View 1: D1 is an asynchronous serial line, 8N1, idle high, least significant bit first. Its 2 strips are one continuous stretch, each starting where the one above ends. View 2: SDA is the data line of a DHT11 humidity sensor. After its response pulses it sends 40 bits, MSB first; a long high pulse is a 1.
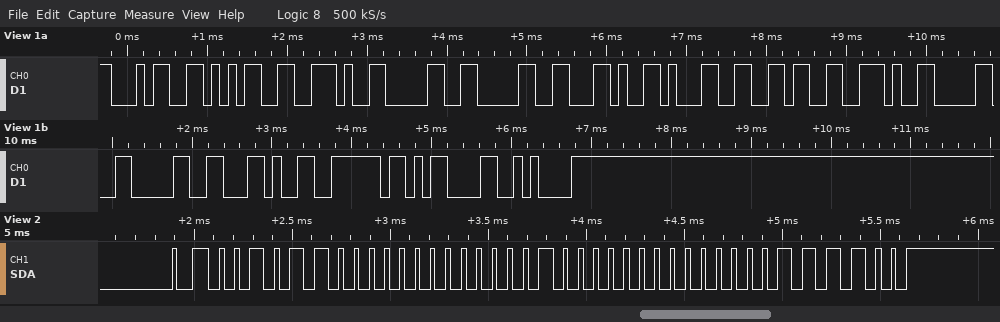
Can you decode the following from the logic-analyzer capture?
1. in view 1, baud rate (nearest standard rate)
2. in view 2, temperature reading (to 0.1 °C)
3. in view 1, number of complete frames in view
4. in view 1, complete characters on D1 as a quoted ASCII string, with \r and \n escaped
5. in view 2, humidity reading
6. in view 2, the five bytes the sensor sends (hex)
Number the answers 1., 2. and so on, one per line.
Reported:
1. 9600 baud
2. 16.0 °C
3. 15
4. "45.00,16.00,~\r\n"
5. 44 %
6. 2C 00 10 00 3C
